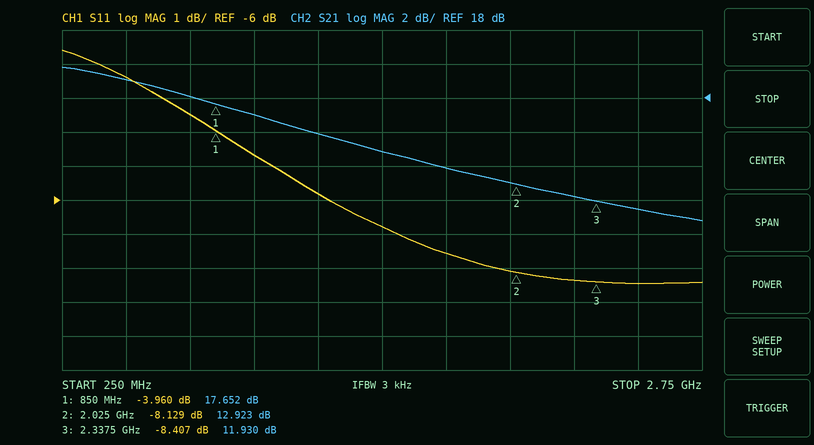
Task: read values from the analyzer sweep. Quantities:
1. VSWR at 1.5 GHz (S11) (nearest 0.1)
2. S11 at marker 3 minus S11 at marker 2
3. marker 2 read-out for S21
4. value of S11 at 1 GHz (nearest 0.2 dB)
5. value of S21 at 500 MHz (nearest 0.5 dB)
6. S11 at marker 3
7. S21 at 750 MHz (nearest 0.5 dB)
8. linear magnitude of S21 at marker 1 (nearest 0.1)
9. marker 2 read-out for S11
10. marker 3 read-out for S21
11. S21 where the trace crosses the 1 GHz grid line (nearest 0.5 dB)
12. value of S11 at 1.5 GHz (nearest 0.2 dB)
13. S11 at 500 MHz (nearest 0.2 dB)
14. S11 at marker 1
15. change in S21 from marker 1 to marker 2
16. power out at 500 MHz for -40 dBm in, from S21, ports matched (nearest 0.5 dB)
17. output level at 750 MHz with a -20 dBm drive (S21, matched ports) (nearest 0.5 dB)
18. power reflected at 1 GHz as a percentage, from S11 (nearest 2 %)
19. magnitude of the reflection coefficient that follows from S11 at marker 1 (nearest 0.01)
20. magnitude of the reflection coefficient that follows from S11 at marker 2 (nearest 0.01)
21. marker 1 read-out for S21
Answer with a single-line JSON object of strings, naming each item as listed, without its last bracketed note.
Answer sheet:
{"VSWR at 1.5 GHz (S11)": "2.7", "S11 at marker 3 minus S11 at marker 2": "-0.278 dB", "marker 2 read-out for S21": "12.923 dB", "value of S11 at 1 GHz": "-4.6 dB", "value of S21 at 500 MHz": "19.0 dB", "S11 at marker 3": "-8.407 dB", "S21 at 750 MHz": "18.0 dB", "linear magnitude of S21 at marker 1": "7.6", "marker 2 read-out for S11": "-8.129 dB", "marker 3 read-out for S21": "11.930 dB", "S21 where the trace crosses the 1 GHz grid line": "17.0 dB", "value of S11 at 1.5 GHz": "-6.8 dB", "S11 at 500 MHz": "-2.4 dB", "S11 at marker 1": "-3.960 dB", "change in S21 from marker 1 to marker 2": "-4.729 dB", "power out at 500 MHz for -40 dBm in, from S21, ports matched": "-21.0 dBm", "output level at 750 MHz with a -20 dBm drive (S21, matched ports)": "-2.0 dBm", "power reflected at 1 GHz as a percentage, from S11": "34 %", "magnitude of the reflection coefficient that follows from S11 at marker 1": "0.63", "magnitude of the reflection coefficient that follows from S11 at marker 2": "0.39", "marker 1 read-out for S21": "17.652 dB"}
